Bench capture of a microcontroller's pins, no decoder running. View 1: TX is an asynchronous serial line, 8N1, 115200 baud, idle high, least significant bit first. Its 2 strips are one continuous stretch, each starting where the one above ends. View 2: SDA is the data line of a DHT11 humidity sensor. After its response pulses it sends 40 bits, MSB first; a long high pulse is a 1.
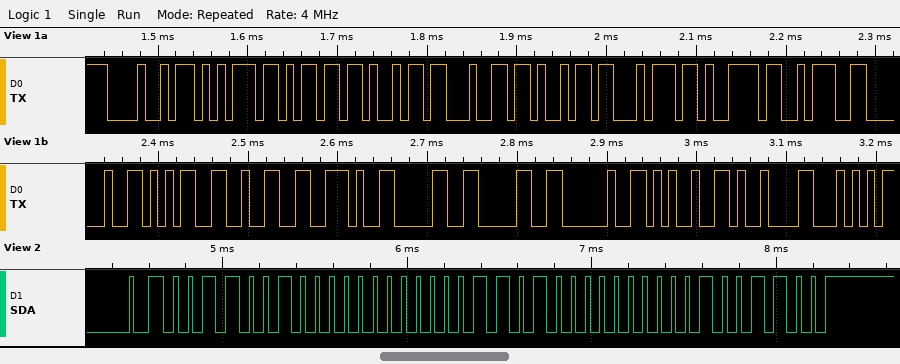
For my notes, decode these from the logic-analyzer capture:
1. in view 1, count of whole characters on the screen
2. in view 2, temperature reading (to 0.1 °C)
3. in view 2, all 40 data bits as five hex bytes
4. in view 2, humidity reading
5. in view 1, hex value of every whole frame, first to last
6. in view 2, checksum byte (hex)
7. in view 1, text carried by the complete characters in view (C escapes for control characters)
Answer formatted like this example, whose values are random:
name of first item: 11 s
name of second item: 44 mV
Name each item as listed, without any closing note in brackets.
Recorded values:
in view 1, count of whole characters on the screen: 19
in view 2, temperature reading: 26.0 °C
in view 2, all 40 data bits as five hex bytes: 32 00 1A 00 4C
in view 2, humidity reading: 50 %
in view 1, hex value of every whole frame, first to last: 0x48 0x75 0x6D 0x69 0x64 0x69 0x74 0x79 0x3A 0x20 0x35 0x32 0x2E 0x30 0x30 0x20 0x25 0x09 0x54
in view 2, checksum byte: 0x4C
in view 1, text carried by the complete characters in view: "Humidity: 52.00 %\tT"
